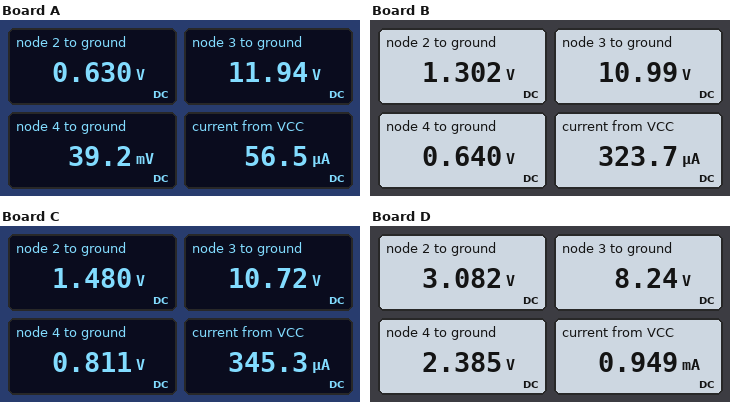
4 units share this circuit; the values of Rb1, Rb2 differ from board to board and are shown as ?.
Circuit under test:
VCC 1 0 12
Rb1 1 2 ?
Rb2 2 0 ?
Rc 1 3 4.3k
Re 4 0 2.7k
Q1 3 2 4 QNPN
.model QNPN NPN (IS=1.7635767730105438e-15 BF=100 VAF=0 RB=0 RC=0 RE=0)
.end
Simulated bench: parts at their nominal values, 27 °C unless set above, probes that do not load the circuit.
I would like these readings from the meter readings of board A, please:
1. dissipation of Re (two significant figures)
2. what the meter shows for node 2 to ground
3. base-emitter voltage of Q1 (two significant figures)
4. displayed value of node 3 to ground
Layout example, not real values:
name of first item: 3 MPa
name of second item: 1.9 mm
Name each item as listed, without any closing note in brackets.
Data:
dissipation of Re: 570 nW
what the meter shows for node 2 to ground: 0.630 V
base-emitter voltage of Q1: 590 mV
displayed value of node 3 to ground: 11.94 V
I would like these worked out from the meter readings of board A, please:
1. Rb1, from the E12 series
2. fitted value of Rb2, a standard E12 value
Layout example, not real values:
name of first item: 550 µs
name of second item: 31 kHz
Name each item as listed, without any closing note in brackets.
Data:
Rb1, from the E12 series: 270 kΩ
fitted value of Rb2, a standard E12 value: 15 kΩ
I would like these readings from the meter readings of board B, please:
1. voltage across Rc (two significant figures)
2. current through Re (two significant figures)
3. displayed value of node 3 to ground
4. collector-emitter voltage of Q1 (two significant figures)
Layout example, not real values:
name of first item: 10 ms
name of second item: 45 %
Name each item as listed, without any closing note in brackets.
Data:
voltage across Rc: 1.0 V
current through Re: 240 µA
displayed value of node 3 to ground: 10.99 V
collector-emitter voltage of Q1: 10 V
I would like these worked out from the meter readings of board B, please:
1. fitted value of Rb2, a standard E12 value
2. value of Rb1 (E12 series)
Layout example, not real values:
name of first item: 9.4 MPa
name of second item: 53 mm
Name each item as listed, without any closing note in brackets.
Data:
fitted value of Rb2, a standard E12 value: 15 kΩ
value of Rb1: 120 kΩ
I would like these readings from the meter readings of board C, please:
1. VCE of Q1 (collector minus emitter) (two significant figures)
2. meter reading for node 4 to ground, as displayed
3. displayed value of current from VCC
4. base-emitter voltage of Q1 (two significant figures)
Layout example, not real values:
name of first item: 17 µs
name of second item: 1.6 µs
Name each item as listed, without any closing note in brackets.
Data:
VCE of Q1 (collector minus emitter): 9.9 V
meter reading for node 4 to ground, as displayed: 0.811 V
displayed value of current from VCC: 345.3 µA
base-emitter voltage of Q1: 670 mV
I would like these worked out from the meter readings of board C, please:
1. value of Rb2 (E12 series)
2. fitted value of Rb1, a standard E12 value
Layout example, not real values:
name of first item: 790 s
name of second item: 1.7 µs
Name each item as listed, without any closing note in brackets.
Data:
value of Rb2: 33 kΩ
fitted value of Rb1, a standard E12 value: 220 kΩ
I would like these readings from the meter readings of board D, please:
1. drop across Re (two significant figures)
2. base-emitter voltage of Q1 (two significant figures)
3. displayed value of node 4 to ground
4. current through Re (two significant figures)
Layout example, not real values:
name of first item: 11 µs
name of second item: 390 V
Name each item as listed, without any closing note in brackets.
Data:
drop across Re: 2.4 V
base-emitter voltage of Q1: 700 mV
displayed value of node 4 to ground: 2.385 V
current through Re: 880 µA
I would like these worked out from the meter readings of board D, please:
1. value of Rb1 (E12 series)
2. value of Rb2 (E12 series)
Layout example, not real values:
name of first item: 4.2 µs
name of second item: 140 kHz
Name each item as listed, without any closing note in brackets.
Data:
value of Rb1: 120 kΩ
value of Rb2: 47 kΩ
